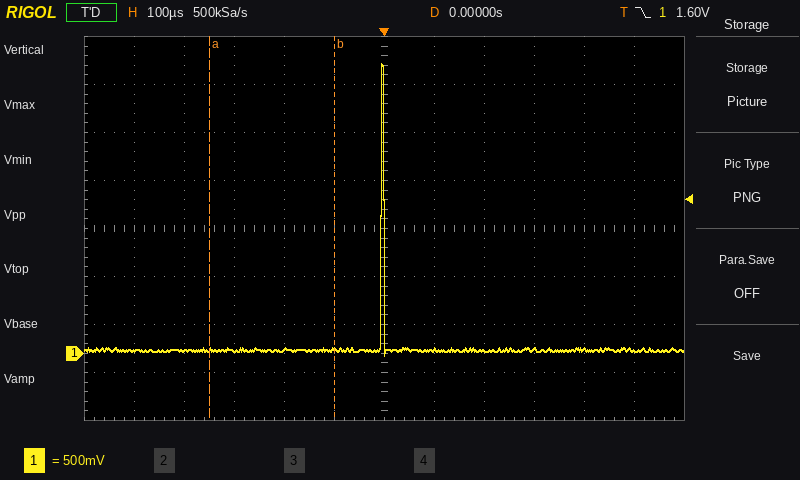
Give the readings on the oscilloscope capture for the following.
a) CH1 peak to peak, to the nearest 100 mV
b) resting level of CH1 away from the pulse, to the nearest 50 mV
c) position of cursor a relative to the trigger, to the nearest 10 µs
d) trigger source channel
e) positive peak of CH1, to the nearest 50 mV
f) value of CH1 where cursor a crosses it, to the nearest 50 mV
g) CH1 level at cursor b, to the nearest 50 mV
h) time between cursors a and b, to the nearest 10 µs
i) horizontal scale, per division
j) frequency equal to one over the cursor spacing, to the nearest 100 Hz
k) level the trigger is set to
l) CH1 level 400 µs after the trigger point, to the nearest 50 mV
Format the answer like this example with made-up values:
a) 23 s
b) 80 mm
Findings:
a) 3.00 V
b) 50 mV
c) -350 µs
d) CH1
e) 3.00 V
f) 50 mV
g) 50 mV
h) 250 µs
i) 100 µs
j) 4.0 kHz
k) 1.60 V
l) 50 mV
